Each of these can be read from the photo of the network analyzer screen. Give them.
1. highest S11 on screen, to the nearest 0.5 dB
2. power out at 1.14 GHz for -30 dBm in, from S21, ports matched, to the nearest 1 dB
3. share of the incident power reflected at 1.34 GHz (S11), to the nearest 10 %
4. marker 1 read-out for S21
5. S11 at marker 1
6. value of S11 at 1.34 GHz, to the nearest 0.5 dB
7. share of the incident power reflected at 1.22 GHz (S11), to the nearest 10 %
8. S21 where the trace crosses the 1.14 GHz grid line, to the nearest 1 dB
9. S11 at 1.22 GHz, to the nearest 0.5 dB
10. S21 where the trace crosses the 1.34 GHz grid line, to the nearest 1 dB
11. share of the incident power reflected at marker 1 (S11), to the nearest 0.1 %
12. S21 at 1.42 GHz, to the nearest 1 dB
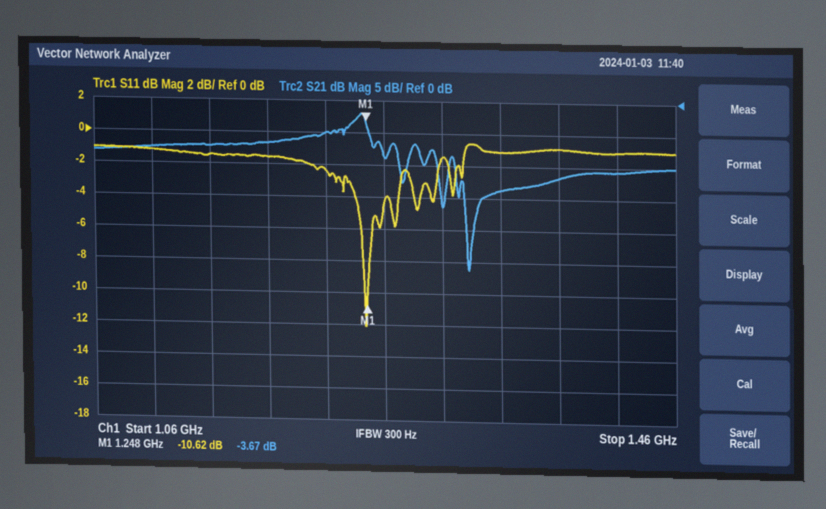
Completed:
-0.5 dB
-37 dBm
80 %
-3.67 dB
-10.62 dB
-1.0 dB
60 %
-7 dB
-2.5 dB
-14 dB
8.7 %
-11 dB
